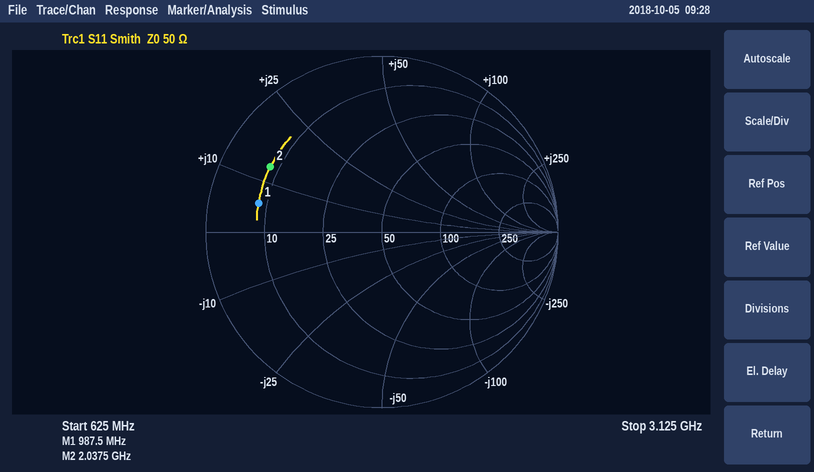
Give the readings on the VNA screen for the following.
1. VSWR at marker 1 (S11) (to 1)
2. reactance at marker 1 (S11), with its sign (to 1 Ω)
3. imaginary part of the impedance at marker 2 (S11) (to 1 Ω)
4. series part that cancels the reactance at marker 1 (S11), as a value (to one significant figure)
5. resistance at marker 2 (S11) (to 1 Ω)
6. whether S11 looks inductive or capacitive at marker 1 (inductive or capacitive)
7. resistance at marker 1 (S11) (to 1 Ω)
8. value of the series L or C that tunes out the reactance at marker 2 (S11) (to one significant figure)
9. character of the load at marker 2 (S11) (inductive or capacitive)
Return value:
6
+6 Ω
+13 Ω
30 pF
8 Ω
inductive
8 Ω
6 pF
inductive
